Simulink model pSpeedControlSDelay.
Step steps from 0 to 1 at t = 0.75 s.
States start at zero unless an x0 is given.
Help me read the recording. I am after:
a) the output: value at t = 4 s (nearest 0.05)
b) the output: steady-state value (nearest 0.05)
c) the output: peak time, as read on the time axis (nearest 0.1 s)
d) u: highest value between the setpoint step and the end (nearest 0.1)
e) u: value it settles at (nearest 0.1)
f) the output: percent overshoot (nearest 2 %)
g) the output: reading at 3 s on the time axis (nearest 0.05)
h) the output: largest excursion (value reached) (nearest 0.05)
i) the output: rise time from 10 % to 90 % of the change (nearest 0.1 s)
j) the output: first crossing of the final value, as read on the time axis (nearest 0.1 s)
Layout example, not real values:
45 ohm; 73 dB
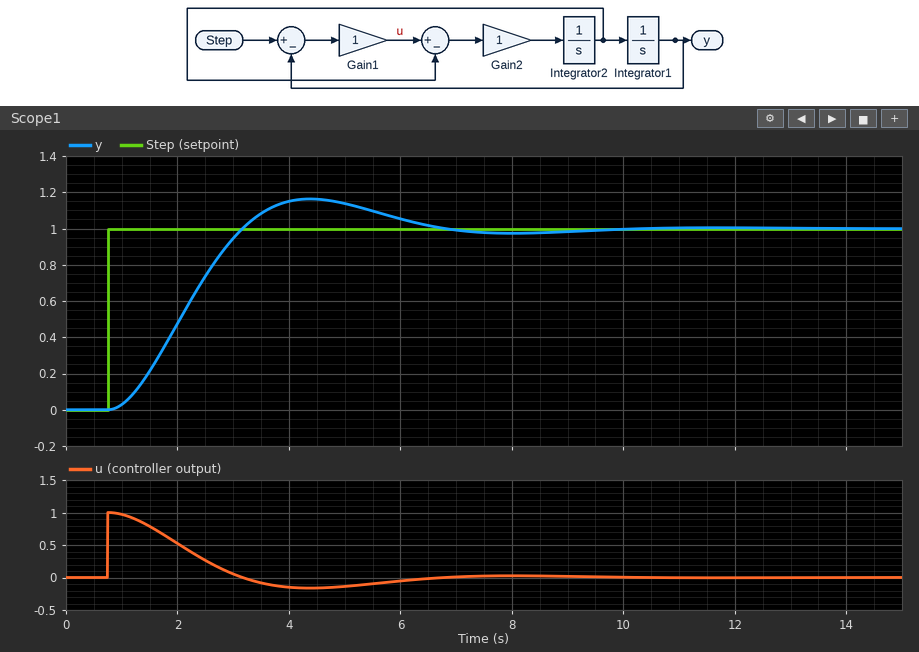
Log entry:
1.15; 1.00; 4.4 s; 1.0; 0.0; 16 %; 0.95; 1.15; 1.6 s; 3.2 s
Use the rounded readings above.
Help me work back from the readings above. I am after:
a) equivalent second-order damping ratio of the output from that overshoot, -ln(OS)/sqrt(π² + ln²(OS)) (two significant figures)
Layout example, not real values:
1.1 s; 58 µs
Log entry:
0.50
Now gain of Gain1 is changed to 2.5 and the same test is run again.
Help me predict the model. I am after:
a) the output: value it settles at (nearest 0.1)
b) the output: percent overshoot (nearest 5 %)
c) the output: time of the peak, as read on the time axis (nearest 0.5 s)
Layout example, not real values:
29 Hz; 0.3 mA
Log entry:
1.0; 35 %; 3.0 s
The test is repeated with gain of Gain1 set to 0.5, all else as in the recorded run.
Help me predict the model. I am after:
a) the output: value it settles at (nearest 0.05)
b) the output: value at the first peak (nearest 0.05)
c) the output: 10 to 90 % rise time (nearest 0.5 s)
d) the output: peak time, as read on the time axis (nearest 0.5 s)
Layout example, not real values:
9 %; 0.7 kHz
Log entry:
1.00; 1.05; 3.0 s; 7.0 s
